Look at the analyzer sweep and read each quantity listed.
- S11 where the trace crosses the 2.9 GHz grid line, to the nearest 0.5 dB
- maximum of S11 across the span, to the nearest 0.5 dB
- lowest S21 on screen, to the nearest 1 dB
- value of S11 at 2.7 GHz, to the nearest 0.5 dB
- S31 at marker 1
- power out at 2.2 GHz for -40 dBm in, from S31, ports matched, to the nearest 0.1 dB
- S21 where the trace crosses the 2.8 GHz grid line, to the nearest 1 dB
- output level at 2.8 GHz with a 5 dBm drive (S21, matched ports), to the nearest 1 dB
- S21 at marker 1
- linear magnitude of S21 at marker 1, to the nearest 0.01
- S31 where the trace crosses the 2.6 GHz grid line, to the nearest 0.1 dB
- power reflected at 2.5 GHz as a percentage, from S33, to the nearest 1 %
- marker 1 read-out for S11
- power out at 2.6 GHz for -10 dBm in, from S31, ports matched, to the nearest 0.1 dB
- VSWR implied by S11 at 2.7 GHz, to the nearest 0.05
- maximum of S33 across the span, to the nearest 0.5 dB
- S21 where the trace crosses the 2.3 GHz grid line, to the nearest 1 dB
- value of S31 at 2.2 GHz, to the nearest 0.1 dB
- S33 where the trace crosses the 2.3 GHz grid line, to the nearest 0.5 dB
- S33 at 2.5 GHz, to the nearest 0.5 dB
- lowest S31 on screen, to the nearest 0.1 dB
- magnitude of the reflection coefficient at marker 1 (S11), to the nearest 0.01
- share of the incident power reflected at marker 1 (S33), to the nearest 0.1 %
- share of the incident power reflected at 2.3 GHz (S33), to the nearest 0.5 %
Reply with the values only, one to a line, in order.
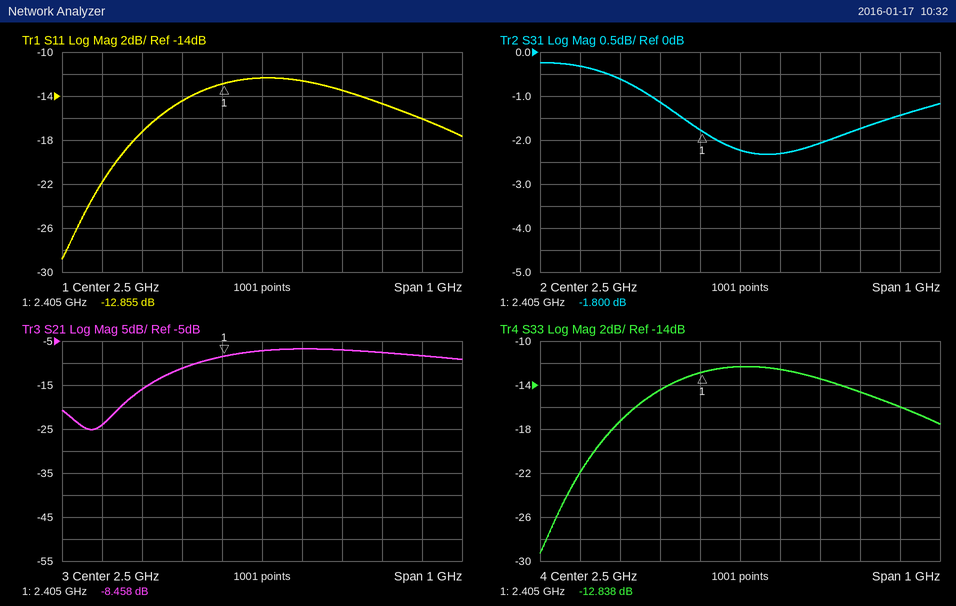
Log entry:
-16.0 dB
-12.5 dB
-25 dB
-13.5 dB
-1.800 dB
-40.6 dBm
-8 dB
-3 dBm
-8.458 dB
0.38
-2.3 dB
6 %
-12.855 dB
-12.3 dBm
1.55
-12.5 dB
-11 dB
-0.6 dB
-14.5 dB
-12.5 dB
-2.3 dB
0.23
5.2 %
3.5 %
